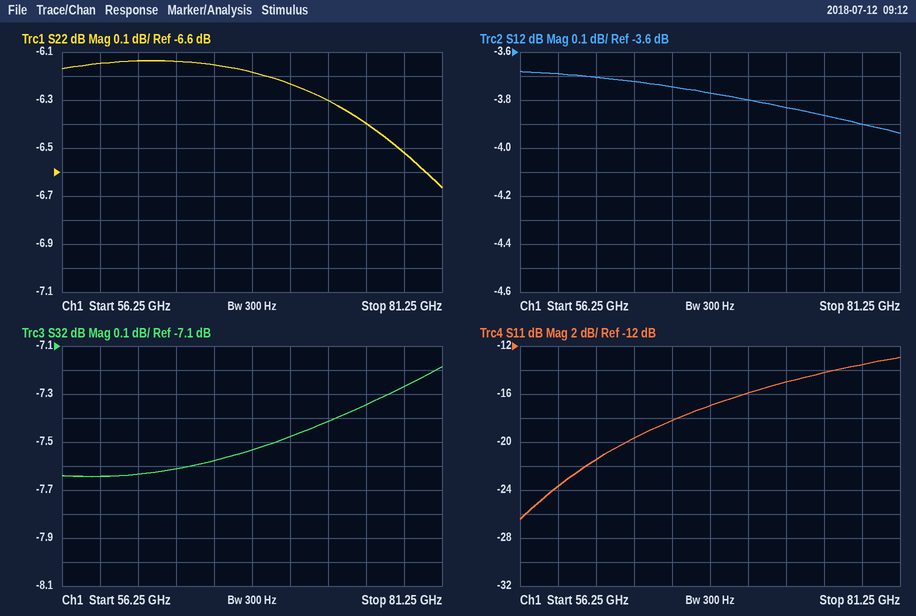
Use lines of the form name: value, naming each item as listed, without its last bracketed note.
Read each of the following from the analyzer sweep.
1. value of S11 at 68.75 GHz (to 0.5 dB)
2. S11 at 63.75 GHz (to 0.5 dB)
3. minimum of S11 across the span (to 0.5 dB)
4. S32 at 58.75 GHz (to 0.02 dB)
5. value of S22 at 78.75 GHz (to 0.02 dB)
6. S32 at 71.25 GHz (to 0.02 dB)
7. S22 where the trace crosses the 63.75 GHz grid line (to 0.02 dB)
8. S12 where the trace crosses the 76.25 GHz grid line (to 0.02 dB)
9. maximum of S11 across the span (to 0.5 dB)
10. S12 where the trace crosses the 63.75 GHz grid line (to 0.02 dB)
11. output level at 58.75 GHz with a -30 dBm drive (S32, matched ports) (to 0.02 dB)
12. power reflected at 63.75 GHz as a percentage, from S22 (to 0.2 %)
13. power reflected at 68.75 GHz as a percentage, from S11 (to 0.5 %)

value of S11 at 68.75 GHz: -17.0 dB
S11 at 63.75 GHz: -19.5 dB
minimum of S11 across the span: -26.5 dB
S32 at 58.75 GHz: -7.64 dB
value of S22 at 78.75 GHz: -6.52 dB
S32 at 71.25 GHz: -7.48 dB
S22 where the trace crosses the 63.75 GHz grid line: -6.14 dB
S12 where the trace crosses the 76.25 GHz grid line: -3.86 dB
maximum of S11 across the span: -13.0 dB
S12 where the trace crosses the 63.75 GHz grid line: -3.72 dB
output level at 58.75 GHz with a -30 dBm drive (S32, matched ports): -37.64 dBm
power reflected at 63.75 GHz as a percentage, from S22: 24.4 %
power reflected at 68.75 GHz as a percentage, from S11: 2.0 %
